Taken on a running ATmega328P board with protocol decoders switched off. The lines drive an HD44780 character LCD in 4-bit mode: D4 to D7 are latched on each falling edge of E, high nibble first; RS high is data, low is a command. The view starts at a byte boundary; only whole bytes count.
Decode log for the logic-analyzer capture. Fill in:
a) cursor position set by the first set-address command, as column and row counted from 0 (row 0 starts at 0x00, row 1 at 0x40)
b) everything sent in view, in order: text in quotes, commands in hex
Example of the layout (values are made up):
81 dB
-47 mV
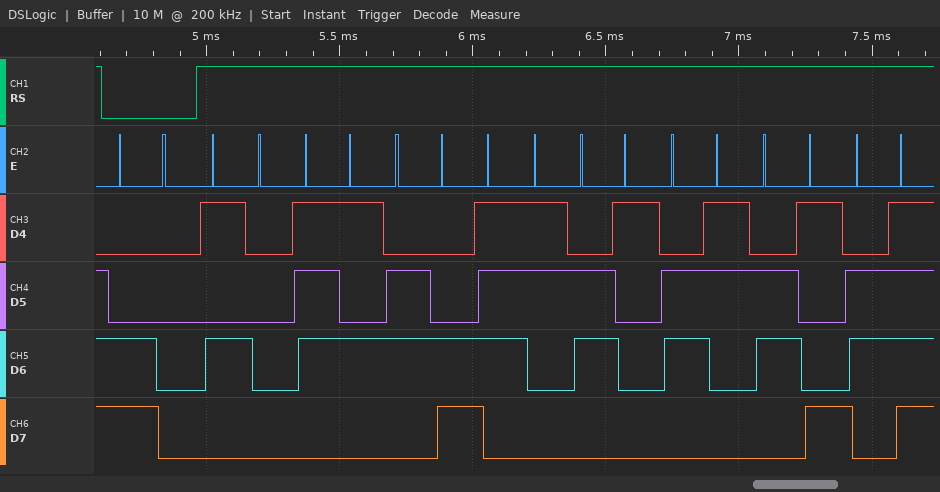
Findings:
column 0, row 1
0xC0 "Pulsacio"
